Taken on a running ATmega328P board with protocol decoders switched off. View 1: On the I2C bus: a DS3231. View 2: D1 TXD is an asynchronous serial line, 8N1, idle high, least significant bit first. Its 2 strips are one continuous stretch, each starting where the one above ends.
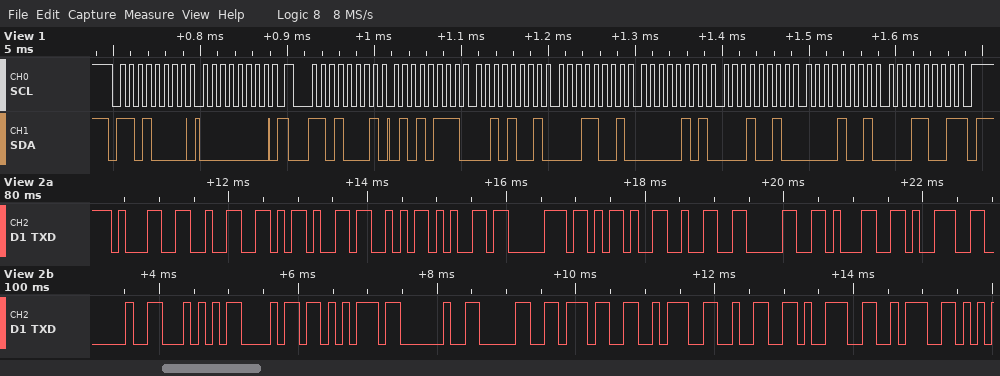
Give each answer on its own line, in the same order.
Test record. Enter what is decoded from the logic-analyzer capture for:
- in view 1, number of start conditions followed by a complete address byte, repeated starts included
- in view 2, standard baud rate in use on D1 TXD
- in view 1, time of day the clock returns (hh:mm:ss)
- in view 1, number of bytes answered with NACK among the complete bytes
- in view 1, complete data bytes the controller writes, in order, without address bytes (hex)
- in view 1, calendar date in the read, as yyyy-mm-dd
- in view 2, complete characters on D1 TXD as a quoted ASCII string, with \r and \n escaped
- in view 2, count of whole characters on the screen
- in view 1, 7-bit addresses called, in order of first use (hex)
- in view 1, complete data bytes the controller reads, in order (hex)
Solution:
2
9600 baud
19:29:57
1
00
2019-09-12
"12-Sep-2019 Thu 07:29:"
22
0x68
57 29 19 05 12 09 19
